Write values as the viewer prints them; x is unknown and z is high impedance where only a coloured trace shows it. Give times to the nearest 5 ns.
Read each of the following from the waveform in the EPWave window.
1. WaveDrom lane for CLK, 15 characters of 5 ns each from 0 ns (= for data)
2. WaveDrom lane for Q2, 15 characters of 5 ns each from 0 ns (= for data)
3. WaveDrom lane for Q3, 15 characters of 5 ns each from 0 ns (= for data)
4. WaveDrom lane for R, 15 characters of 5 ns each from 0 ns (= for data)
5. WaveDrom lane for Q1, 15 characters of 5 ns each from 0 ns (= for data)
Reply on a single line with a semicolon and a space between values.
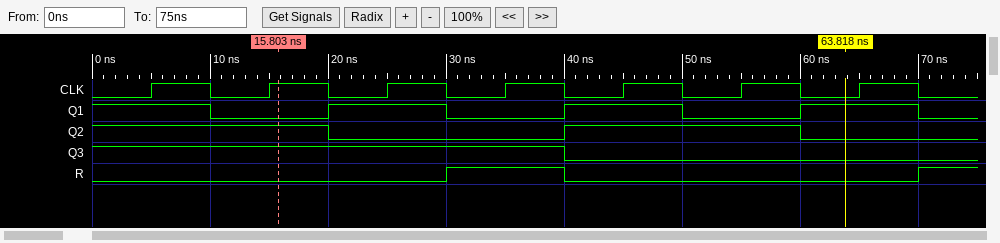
{name: 'CLK', wave: '010101010101010'}; {name: 'Q2', wave: '1...0...1...0..'}; {name: 'Q3', wave: '1.......0......'}; {name: 'R', wave: '0.....1.0.....1'}; {name: 'Q1', wave: '1.0.1.0.1.0.1.0'}
